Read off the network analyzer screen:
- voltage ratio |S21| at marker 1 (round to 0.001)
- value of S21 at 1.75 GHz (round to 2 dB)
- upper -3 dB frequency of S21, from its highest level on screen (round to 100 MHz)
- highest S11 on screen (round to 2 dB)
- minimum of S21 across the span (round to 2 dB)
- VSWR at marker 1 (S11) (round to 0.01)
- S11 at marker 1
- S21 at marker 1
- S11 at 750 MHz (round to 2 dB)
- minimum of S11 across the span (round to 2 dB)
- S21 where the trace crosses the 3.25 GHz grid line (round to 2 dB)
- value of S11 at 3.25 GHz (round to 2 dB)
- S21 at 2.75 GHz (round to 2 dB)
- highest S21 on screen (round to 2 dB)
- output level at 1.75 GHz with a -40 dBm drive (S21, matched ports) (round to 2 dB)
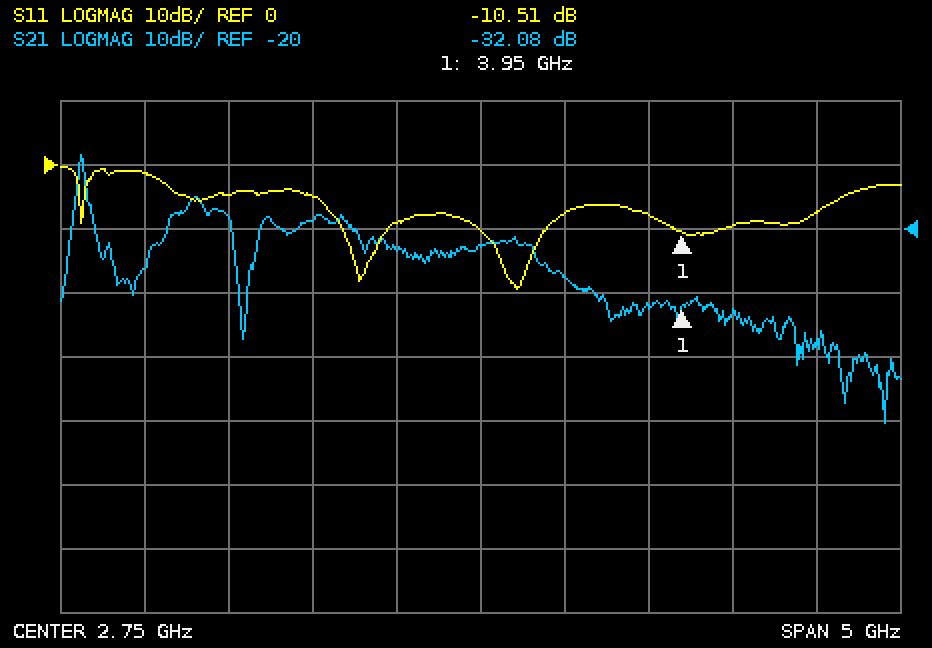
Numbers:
0.025
-18 dB
400 MHz
0 dB
-50 dB
1.85
-10.51 dB
-32.08 dB
-2 dB
-20 dB
-28 dB
-8 dB
-22 dB
-8 dB
-58 dBm
